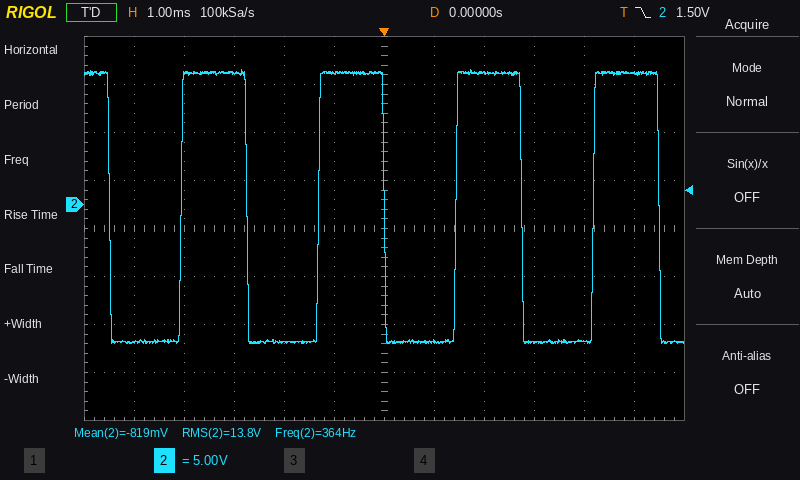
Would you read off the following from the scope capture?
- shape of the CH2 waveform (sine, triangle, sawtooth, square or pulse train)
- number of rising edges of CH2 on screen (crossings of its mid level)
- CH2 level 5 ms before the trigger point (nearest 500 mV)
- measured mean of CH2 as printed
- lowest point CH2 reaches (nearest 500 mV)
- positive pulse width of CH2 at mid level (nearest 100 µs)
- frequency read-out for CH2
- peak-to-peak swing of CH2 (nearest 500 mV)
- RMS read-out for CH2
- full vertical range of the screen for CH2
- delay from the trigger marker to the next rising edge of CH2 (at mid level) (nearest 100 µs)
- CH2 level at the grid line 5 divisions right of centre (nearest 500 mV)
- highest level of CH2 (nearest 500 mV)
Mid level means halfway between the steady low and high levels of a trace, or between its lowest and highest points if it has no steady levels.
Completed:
square
4
-14.5 V
-819 mV
-14.5 V
1.3 ms
364 Hz
28.5 V
13.8 V
40 V
1.4 ms
13.5 V
14.0 V
